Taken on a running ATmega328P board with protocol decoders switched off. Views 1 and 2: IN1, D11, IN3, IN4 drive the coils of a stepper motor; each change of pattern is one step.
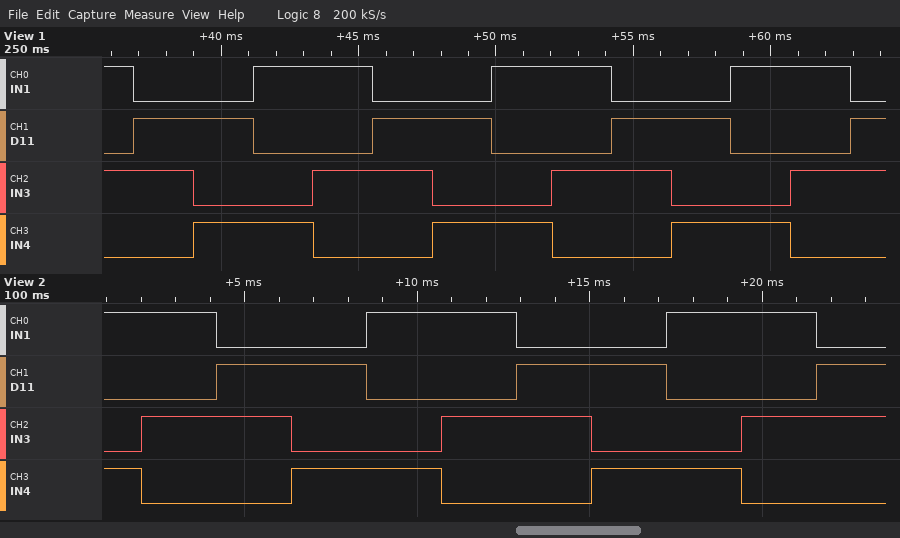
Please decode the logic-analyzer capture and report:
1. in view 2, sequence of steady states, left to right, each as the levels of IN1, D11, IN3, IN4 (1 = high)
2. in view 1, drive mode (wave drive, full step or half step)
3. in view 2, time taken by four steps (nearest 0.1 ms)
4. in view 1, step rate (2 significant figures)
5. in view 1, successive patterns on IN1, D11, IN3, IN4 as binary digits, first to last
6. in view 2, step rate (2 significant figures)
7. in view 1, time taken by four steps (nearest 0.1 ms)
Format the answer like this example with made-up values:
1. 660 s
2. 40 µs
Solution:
1. 1001 1010 0110 0101 1001 1010 0110 0101 1001 1010 0110
2. full step
3. 8.7 ms
4. 460 steps/s
5. 1010 0110 0101 1001 1010 0110 0101 1001 1010 0110 0101 1001 1010 0110
6. 460 steps/s
7. 8.7 ms
